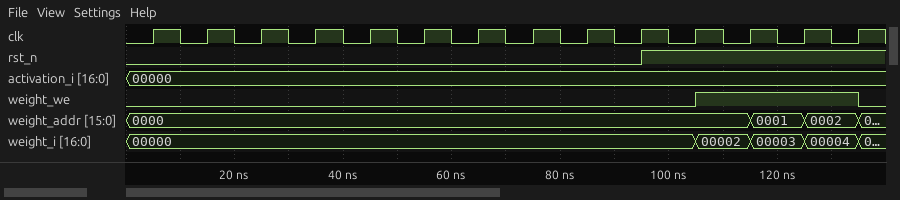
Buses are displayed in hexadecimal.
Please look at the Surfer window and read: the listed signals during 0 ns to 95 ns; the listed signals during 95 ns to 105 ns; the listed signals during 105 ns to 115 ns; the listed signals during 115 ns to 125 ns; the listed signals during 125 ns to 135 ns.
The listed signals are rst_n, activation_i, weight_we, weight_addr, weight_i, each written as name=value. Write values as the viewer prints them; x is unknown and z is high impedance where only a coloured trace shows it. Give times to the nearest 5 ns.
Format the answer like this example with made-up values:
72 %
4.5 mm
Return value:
rst_n=0, activation_i=00000, weight_we=0, weight_addr=0000, weight_i=00000
rst_n=1, activation_i=00000, weight_we=0, weight_addr=0000, weight_i=00000
rst_n=1, activation_i=00000, weight_we=1, weight_addr=0000, weight_i=00002
rst_n=1, activation_i=00000, weight_we=1, weight_addr=0001, weight_i=00003
rst_n=1, activation_i=00000, weight_we=1, weight_addr=0002, weight_i=00004
